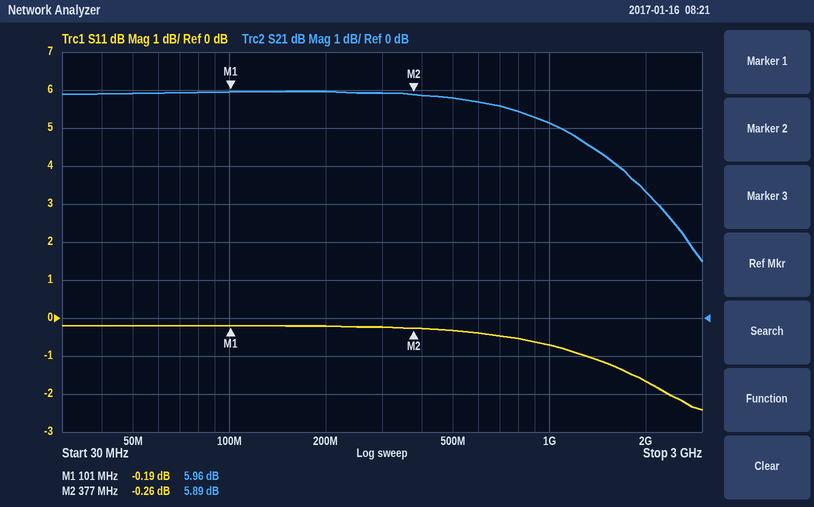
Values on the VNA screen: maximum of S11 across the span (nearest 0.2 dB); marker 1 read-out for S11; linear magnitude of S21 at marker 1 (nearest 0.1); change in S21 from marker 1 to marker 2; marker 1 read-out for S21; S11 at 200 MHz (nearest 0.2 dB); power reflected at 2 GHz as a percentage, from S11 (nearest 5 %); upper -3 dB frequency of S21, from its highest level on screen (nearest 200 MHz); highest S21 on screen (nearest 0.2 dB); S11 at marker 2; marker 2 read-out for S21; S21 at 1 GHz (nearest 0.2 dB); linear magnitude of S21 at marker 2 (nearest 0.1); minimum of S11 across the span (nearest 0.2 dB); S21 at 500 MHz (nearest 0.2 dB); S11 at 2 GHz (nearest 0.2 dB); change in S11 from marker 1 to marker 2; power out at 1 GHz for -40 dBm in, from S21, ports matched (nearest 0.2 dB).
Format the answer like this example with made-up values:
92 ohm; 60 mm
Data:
-0.2 dB; -0.19 dB; 2.0; -0.07 dB; 5.96 dB; -0.2 dB; 70 %; 2.2 GHz; 6.0 dB; -0.26 dB; 5.89 dB; 5.2 dB; 2.0; -2.4 dB; 5.8 dB; -1.6 dB; -0.07 dB; -34.8 dBm
